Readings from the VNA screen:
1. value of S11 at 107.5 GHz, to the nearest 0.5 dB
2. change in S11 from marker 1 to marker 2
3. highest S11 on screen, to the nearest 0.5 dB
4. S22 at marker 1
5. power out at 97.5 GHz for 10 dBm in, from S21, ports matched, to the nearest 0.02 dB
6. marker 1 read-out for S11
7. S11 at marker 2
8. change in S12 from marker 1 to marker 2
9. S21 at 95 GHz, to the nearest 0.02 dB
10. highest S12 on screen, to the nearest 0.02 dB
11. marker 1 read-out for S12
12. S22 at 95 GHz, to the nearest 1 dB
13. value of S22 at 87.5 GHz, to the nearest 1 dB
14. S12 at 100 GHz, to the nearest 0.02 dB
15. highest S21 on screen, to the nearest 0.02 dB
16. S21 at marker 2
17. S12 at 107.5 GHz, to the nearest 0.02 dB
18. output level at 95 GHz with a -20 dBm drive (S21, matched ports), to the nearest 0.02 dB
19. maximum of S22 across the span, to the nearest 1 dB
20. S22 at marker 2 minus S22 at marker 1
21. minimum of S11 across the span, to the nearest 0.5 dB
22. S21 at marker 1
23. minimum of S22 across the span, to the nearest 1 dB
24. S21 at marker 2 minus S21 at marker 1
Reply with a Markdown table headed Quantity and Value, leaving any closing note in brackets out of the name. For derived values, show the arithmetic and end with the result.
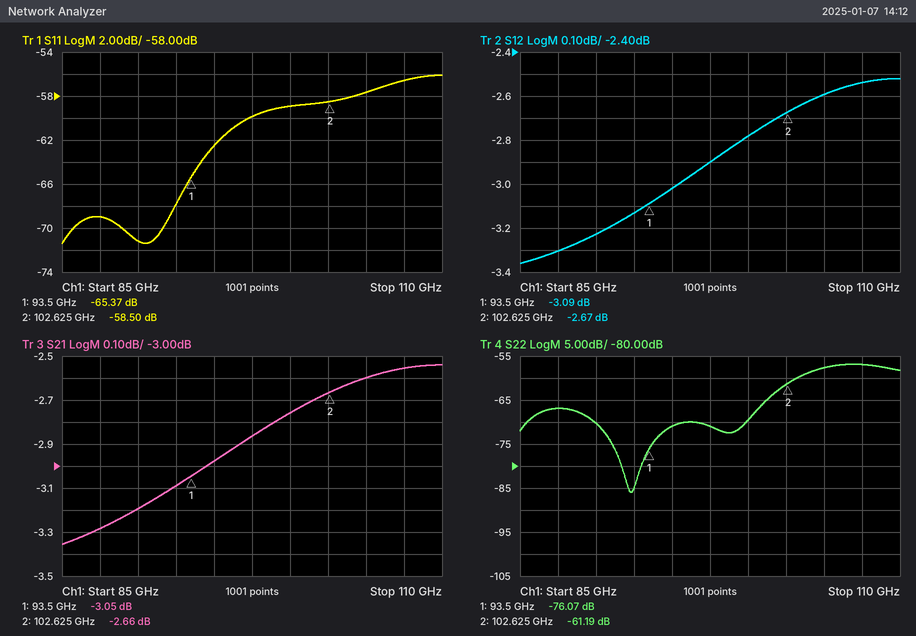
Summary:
| Quantity | Value |
|---|---|
| value of S11 at 107.5 GHz, to the nearest 0.5 dB | -56.5 dB |
| change in S11 from marker 1 to marker 2 | -58.5 − (-65.37) = 6.87 dB |
| highest S11 on screen, to the nearest 0.5 dB | -56.0 dB |
| S22 at marker 1 | -76.07 dB |
| power out at 97.5 GHz for 10 dBm in, from S21, ports matched, to the nearest 0.02 dB | 10 dBm + (-2.86 dB) = 7.14 dBm |
| marker 1 read-out for S11 | -65.37 dB |
| S11 at marker 2 | -58.50 dB |
| change in S12 from marker 1 to marker 2 | -2.67 − (-3.09) = 0.42 dB |
| S21 at 95 GHz, to the nearest 0.02 dB | -2.98 dB |
| highest S12 on screen, to the nearest 0.02 dB | -2.52 dB |
| marker 1 read-out for S12 | -3.09 dB |
| S22 at 95 GHz, to the nearest 1 dB | -71 dB |
| value of S22 at 87.5 GHz, to the nearest 1 dB | -67 dB |
| S12 at 100 GHz, to the nearest 0.02 dB | -2.78 dB |
| highest S21 on screen, to the nearest 0.02 dB | -2.54 dB |
| S21 at marker 2 | -2.66 dB |
| S12 at 107.5 GHz, to the nearest 0.02 dB | -2.54 dB |
| output level at 95 GHz with a -20 dBm drive (S21, matched ports), to the nearest 0.02 dB | -20 dBm + (-2.98 dB) = -22.98 dBm |
| maximum of S22 across the span, to the nearest 1 dB | -57 dB |
| S22 at marker 2 minus S22 at marker 1 | -61.19 − (-76.07) = 14.88 dB |
| minimum of S11 across the span, to the nearest 0.5 dB | -71.5 dB |
| S21 at marker 1 | -3.05 dB |
| minimum of S22 across the span, to the nearest 1 dB | -86 dB |
| S21 at marker 2 minus S21 at marker 1 | -2.66 − (-3.05) = 0.39 dB |
